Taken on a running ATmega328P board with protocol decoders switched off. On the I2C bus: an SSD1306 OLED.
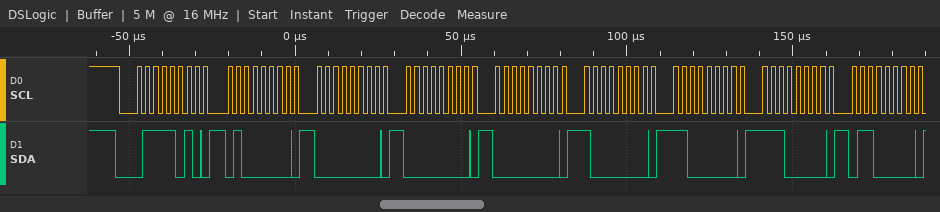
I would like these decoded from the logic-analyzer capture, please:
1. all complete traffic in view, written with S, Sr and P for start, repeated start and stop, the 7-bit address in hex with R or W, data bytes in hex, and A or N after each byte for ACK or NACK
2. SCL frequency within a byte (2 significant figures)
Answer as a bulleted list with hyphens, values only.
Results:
- S 3DW A 40 A 00 A 00 A 00 A 80 A C0 A E0 A 60 A
- 400 kHz
